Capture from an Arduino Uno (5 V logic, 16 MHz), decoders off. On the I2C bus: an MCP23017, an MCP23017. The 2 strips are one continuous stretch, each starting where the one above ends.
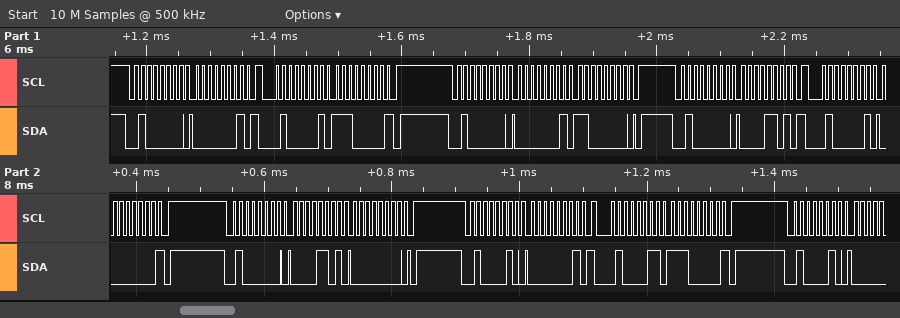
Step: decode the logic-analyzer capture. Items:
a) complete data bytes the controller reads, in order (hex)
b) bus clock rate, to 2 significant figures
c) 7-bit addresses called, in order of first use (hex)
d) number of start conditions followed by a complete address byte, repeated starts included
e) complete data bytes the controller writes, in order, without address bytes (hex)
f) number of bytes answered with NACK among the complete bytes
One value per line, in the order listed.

E0 00 E0
100 kHz
0x20 0x21
9
01 01 C0 0D 0D 00 01
3
